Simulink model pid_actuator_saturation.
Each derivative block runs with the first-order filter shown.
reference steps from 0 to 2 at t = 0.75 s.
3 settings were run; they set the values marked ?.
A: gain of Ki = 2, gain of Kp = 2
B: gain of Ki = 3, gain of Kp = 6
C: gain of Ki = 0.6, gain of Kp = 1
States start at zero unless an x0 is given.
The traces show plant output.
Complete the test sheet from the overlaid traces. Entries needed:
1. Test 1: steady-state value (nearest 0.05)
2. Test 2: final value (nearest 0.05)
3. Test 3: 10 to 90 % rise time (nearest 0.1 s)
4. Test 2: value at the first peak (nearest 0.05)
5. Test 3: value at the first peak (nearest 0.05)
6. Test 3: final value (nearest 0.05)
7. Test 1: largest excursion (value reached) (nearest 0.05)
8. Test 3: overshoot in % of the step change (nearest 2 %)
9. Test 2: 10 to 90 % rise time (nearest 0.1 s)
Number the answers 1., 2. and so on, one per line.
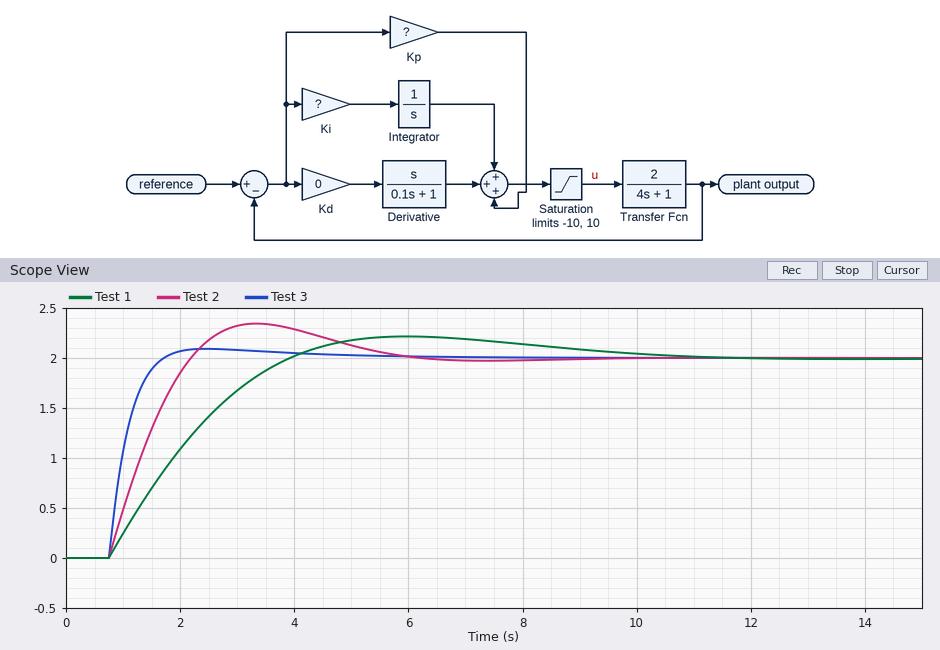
1. 2.00
2. 2.00
3. 0.6 s
4. 2.35
5. 2.10
6. 2.00
7. 2.20
8. 4 %
9. 1.1 s
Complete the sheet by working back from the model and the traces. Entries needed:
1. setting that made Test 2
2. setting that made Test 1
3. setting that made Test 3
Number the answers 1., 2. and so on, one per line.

1. A
2. C
3. B
